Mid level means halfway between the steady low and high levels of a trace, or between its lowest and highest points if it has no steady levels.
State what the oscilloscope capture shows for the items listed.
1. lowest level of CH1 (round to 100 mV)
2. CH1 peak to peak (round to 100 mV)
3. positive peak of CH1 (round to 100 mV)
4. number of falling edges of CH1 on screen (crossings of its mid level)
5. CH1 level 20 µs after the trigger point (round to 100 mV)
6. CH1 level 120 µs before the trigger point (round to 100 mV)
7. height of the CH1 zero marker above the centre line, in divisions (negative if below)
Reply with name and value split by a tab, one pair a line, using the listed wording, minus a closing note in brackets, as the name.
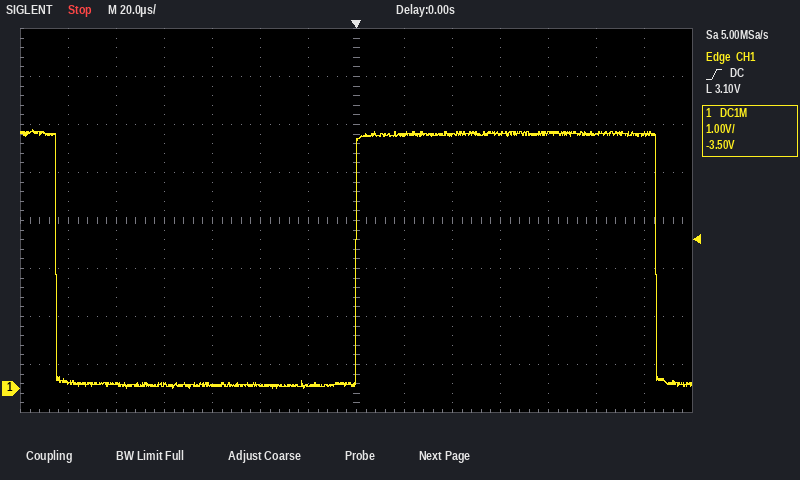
lowest level of CH1	0.0 V
CH1 peak to peak	5.4 V
positive peak of CH1	5.4 V
number of falling edges of CH1 on screen	2
CH1 level 20 µs after the trigger point	5.3 V
CH1 level 120 µs before the trigger point	100 mV
height of the CH1 zero marker above the centre line, in divisions	-3.5 div
